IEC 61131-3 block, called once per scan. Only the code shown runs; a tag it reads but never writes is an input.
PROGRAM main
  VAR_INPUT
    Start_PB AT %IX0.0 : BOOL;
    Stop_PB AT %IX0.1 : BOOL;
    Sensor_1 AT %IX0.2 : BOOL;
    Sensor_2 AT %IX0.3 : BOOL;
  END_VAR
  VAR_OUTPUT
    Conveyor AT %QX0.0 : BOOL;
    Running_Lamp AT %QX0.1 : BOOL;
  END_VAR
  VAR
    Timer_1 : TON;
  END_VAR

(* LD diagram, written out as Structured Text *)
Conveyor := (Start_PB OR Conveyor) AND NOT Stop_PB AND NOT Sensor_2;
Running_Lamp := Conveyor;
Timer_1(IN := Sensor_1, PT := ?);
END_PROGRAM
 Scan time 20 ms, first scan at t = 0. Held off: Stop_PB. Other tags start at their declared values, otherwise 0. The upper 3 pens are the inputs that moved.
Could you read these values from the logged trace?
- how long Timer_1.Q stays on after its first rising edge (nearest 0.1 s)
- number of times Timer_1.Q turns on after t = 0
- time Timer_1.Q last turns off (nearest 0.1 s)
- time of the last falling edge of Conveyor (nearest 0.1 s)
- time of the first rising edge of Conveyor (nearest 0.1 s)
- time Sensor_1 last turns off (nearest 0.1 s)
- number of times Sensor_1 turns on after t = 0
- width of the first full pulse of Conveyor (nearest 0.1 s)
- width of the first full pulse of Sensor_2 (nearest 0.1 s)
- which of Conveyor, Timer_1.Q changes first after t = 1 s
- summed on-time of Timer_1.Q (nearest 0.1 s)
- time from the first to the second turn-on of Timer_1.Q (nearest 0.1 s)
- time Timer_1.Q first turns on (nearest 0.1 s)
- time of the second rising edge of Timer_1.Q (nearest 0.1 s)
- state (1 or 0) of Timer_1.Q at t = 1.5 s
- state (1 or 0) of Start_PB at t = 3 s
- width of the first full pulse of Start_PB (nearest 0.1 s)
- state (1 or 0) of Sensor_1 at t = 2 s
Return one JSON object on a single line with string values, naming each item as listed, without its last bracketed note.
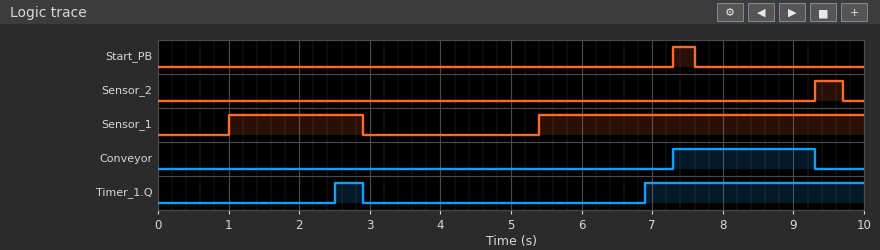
{"how long Timer_1.Q stays on after its first rising edge": "0.4 s", "number of times Timer_1.Q turns on after t = 0": "2", "time Timer_1.Q last turns off": "2.9 s", "time of the last falling edge of Conveyor": "9.3 s", "time of the first rising edge of Conveyor": "7.3 s", "time Sensor_1 last turns off": "2.9 s", "number of times Sensor_1 turns on after t = 0": "2", "width of the first full pulse of Conveyor": "2.0 s", "width of the first full pulse of Sensor_2": "0.4 s", "which of Conveyor, Timer_1.Q changes first after t = 1 s": "Timer_1.Q", "summed on-time of Timer_1.Q": "3.5 s", "time from the first to the second turn-on of Timer_1.Q": "4.4 s", "time Timer_1.Q first turns on": "2.5 s", "time of the second rising edge of Timer_1.Q": "6.9 s", "state (1 or 0) of Timer_1.Q at t = 1.5 s": "0", "state (1 or 0) of Start_PB at t = 3 s": "0", "width of the first full pulse of Start_PB": "0.3 s", "state (1 or 0) of Sensor_1 at t = 2 s": "1"}
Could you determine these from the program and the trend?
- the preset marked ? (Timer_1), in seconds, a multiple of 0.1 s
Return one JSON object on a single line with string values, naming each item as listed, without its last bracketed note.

{"the preset marked ? (Timer_1), in seconds, a multiple of 0.1 s": "1.5 s"}
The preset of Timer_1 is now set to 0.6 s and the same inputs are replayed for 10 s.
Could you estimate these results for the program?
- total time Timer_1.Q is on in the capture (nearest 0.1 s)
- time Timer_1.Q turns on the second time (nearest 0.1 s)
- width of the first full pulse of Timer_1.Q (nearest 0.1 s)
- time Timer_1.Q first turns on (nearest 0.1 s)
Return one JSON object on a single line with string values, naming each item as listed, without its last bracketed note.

{"total time Timer_1.Q is on in the capture": "5.3 s", "time Timer_1.Q turns on the second time": "6.0 s", "width of the first full pulse of Timer_1.Q": "1.3 s", "time Timer_1.Q first turns on": "1.6 s"}
